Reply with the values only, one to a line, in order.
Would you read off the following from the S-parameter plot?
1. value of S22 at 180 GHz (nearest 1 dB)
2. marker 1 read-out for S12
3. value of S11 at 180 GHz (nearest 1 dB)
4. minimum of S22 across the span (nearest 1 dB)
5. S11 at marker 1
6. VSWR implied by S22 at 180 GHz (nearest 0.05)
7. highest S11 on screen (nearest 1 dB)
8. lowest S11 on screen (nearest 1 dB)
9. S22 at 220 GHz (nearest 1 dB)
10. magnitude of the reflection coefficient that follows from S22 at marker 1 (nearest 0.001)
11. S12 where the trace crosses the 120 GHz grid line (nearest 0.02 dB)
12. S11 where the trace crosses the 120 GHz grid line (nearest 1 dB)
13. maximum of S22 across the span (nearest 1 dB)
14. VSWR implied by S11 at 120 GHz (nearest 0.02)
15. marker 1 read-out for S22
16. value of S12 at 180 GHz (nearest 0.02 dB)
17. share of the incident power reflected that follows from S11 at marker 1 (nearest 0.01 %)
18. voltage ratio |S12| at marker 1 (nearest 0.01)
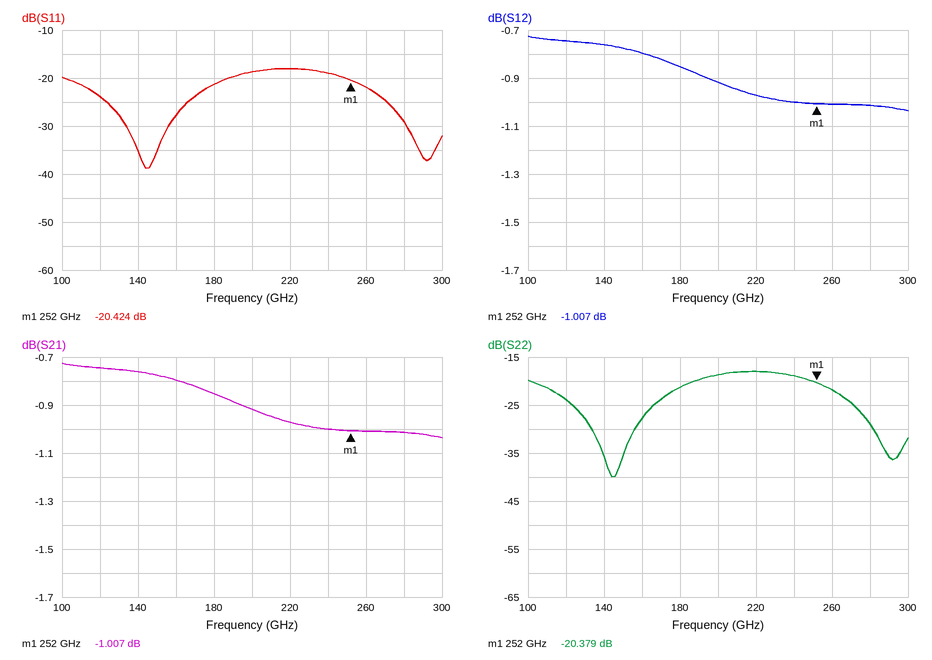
-21 dB
-1.007 dB
-21 dB
-40 dB
-20.424 dB
1.20
-18 dB
-39 dB
-18 dB
0.096
-0.74 dB
-24 dB
-18 dB
1.14
-20.379 dB
-0.86 dB
0.91 %
0.89
